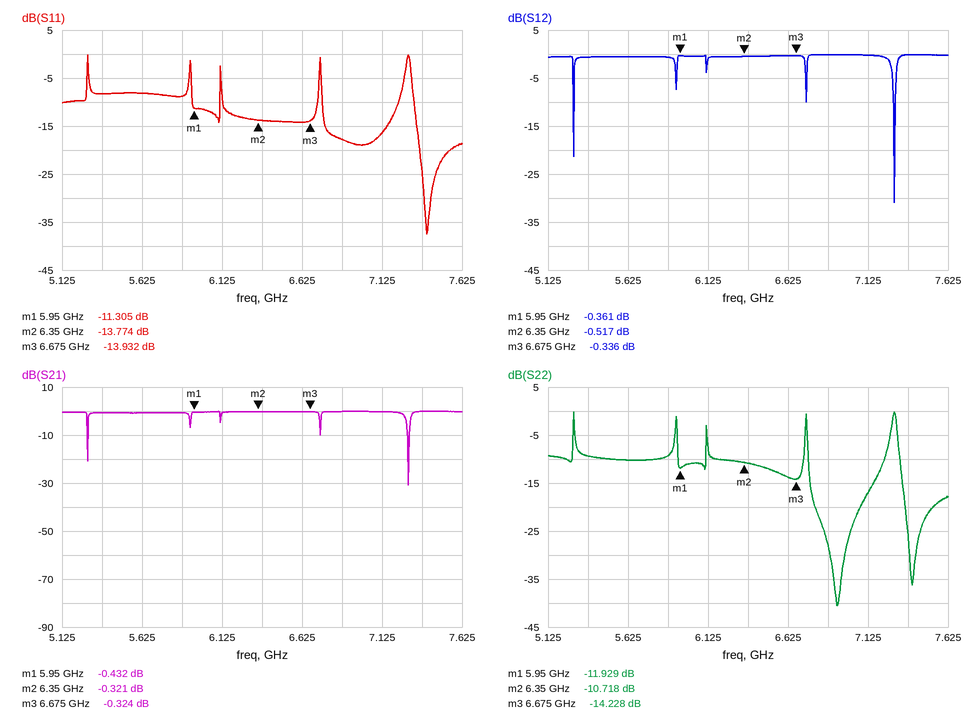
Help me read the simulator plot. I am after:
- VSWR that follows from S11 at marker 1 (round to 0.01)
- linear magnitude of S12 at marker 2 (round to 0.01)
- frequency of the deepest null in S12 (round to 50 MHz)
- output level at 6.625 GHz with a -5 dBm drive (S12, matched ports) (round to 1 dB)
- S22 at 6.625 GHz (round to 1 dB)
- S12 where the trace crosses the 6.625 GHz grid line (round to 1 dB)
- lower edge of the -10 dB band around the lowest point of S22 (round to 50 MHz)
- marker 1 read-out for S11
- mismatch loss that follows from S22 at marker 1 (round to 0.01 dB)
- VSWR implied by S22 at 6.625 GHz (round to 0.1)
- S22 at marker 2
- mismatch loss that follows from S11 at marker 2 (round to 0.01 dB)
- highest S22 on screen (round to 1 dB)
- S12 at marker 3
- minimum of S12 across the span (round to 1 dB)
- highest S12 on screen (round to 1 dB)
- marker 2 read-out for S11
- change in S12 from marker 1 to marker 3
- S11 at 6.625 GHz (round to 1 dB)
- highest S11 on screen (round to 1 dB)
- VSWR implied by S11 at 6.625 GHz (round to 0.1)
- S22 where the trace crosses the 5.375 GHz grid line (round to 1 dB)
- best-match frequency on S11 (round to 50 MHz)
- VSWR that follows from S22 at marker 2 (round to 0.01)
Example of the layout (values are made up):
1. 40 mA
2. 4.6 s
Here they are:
1. 1.75
2. 0.94
3. 7.30 GHz
4. -5 dBm
5. -14 dB
6. 0 dB
7. 6.75 GHz
8. -11.305 dB
9. 0.29 dB
10. 1.5
11. -10.718 dB
12. 0.19 dB
13. 0 dB
14. -0.336 dB
15. -31 dB
16. 0 dB
17. -13.774 dB
18. 0.025 dB
19. -14 dB
20. 0 dB
21. 1.5
22. -9 dB
23. 7.40 GHz
24. 1.82
